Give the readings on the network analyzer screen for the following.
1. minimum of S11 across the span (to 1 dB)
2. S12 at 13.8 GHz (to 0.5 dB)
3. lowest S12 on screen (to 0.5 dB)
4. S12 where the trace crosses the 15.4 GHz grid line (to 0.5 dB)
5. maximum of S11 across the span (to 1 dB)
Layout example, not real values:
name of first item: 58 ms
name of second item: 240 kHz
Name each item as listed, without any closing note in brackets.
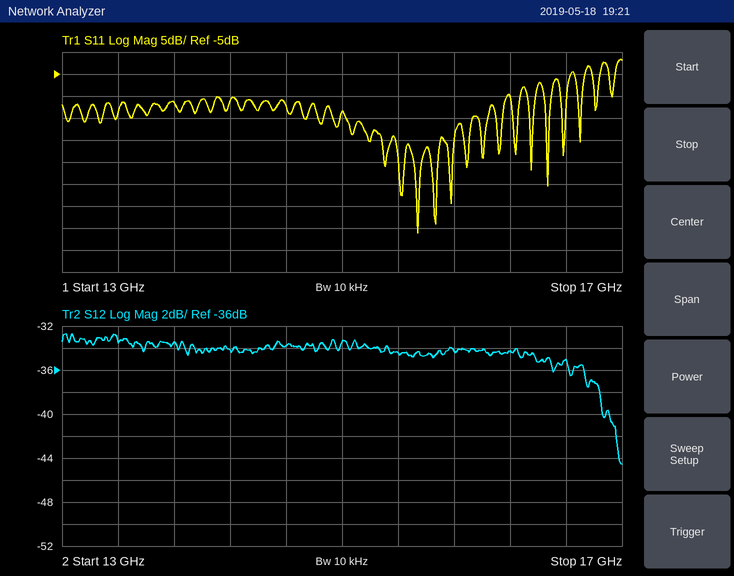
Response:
minimum of S11 across the span: -41 dB
S12 at 13.8 GHz: -33.5 dB
lowest S12 on screen: -44.5 dB
S12 where the trace crosses the 15.4 GHz grid line: -34.5 dB
maximum of S11 across the span: -2 dB
